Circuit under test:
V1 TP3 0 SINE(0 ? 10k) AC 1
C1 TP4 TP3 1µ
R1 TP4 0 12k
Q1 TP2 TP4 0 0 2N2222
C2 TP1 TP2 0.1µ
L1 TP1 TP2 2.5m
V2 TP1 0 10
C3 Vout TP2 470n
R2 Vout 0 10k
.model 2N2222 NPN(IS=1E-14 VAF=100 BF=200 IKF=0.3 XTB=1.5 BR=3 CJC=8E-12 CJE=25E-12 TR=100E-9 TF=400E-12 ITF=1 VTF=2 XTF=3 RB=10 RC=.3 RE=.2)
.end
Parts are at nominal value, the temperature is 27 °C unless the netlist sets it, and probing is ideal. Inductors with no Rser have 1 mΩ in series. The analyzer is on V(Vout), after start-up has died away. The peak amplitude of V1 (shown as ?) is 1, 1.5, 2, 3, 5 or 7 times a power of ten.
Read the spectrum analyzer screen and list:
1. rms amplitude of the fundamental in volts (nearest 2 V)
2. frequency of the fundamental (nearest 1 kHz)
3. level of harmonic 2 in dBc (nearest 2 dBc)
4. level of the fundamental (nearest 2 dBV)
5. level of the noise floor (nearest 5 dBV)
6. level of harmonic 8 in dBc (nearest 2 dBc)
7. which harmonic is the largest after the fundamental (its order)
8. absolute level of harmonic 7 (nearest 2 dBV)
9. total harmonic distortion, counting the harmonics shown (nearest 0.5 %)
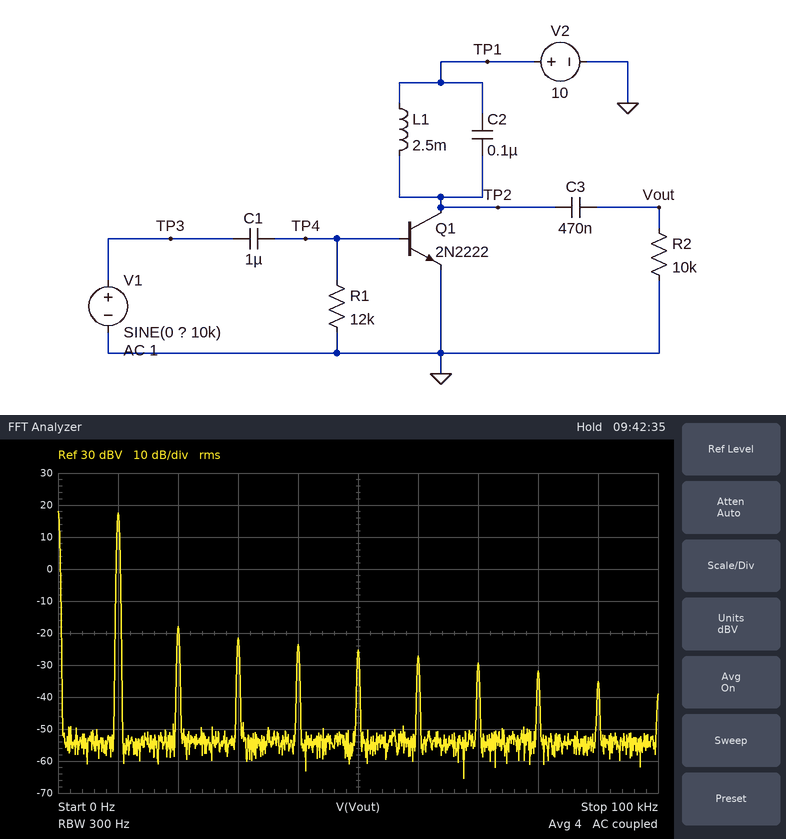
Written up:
8 V
10 kHz
-36 dBc
18 dBV
-55 dBV
-50 dBc
2
-30 dBV
2.5 %
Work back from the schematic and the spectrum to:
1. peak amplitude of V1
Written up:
2 V
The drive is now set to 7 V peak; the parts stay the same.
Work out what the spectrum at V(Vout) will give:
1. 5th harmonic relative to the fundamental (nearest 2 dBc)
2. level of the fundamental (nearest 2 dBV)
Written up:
-42 dBc
18 dBV
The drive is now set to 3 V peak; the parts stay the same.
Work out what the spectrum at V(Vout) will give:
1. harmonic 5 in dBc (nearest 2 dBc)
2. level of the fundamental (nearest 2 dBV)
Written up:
-42 dBc
18 dBV
